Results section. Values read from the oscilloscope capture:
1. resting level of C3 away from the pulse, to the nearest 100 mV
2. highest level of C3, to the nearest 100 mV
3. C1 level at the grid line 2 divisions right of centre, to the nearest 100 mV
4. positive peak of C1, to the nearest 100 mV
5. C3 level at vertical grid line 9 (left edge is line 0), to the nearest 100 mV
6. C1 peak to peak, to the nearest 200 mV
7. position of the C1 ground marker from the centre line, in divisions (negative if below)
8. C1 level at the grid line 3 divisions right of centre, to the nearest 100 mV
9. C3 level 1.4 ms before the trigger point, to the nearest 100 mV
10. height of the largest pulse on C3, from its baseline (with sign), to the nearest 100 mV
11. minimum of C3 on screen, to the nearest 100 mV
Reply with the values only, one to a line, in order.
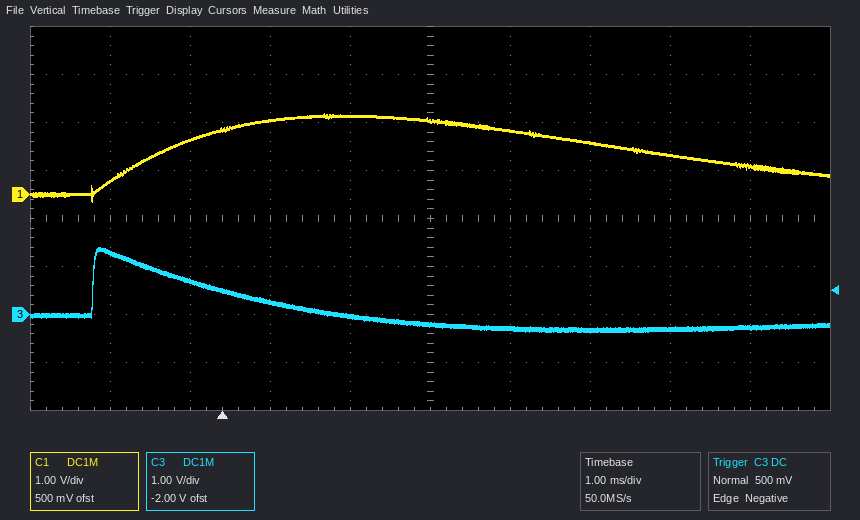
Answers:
-300 mV
1.4 V
1.1 V
1.7 V
-300 mV
1.8 V
+0.5 div
800 mV
1.3 V
+1.7 V
-400 mV
